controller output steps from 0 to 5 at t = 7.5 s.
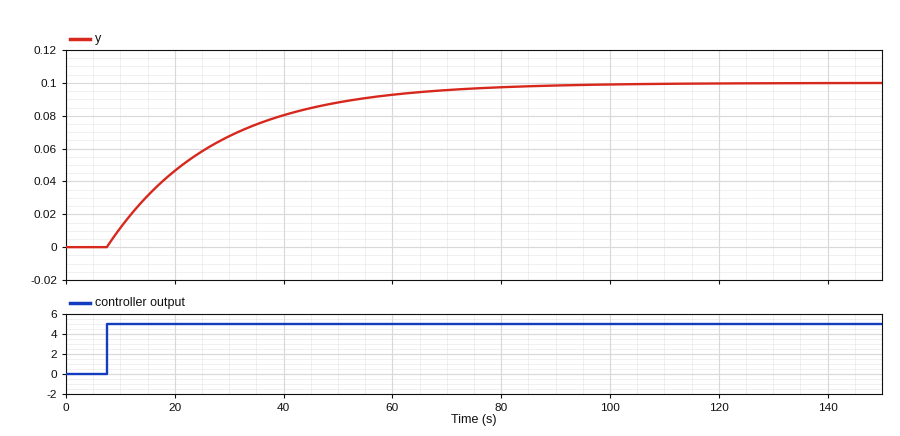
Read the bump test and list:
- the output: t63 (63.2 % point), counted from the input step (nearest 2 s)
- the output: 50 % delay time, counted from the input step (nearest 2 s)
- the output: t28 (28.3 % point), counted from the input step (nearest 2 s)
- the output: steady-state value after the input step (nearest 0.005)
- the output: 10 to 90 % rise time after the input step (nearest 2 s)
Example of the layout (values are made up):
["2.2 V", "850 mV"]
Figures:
["20 s", "14 s", "6 s", "0.100", "44 s"]
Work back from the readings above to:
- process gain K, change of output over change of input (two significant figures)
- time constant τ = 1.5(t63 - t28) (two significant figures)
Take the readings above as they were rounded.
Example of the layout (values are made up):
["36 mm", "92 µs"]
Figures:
["0.020", "21 s"]
